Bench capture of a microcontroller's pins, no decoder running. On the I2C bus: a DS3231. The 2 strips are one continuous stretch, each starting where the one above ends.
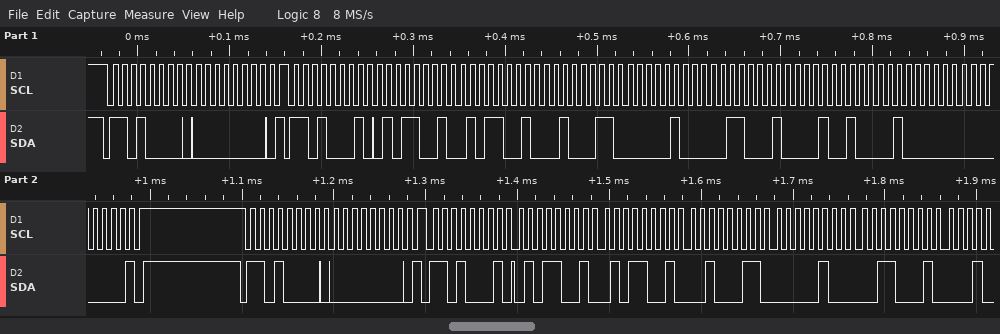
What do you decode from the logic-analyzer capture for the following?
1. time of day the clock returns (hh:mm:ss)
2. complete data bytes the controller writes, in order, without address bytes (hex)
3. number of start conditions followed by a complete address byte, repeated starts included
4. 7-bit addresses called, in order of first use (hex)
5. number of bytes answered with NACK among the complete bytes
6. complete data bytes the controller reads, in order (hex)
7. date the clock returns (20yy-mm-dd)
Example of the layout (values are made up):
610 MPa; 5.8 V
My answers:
23:59:59; 00 00; 4; 0x68; 1; 59 59 23 04 31 12 20 00 59 59 23 04 31; 2020-12-31
